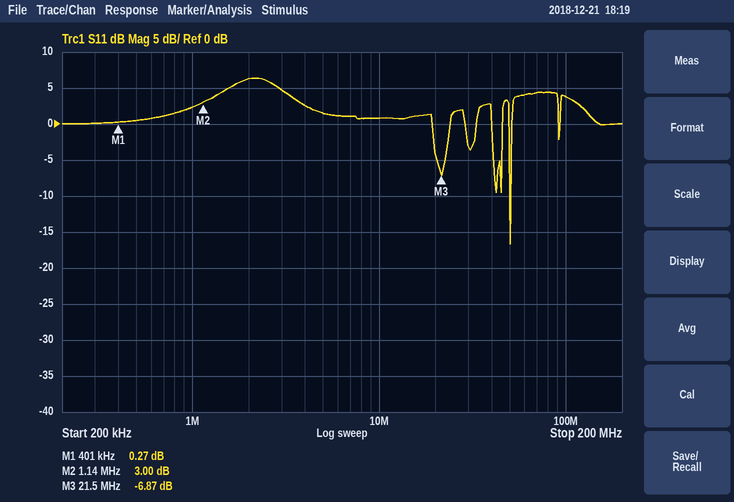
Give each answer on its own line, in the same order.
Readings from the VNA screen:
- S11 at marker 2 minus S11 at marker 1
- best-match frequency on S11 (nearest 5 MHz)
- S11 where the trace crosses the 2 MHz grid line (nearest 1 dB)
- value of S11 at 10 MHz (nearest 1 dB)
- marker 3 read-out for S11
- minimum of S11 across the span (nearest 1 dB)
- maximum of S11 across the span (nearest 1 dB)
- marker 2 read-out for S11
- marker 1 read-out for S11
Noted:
2.73 dB
50 MHz
6 dB
1 dB
-6.87 dB
-17 dB
6 dB
3.00 dB
0.27 dB
